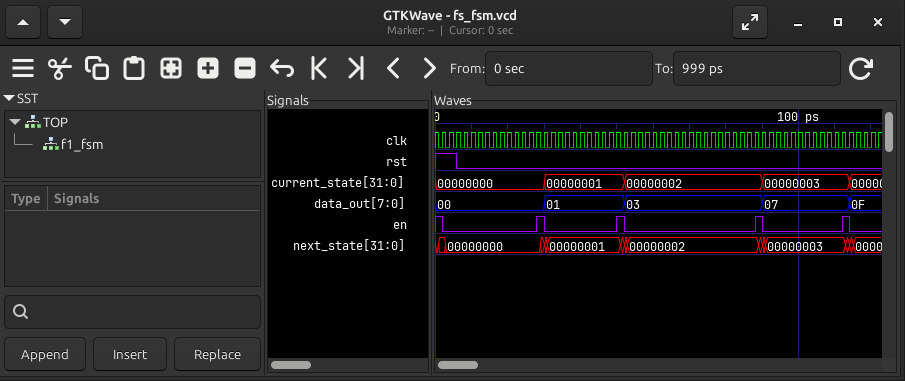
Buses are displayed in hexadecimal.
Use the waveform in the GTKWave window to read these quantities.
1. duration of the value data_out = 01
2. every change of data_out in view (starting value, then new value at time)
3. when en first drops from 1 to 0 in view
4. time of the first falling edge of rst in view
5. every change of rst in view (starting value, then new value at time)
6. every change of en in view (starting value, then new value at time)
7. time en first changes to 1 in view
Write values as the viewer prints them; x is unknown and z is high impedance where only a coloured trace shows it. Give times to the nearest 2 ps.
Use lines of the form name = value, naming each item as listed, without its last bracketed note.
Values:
duration of the value data_out = 01 = 22 ps
every change of data_out in view = 00, 01 at 30 ps, 03 at 52 ps, 07 at 90 ps, 0F at 114 ps
when en first drops from 1 to 0 in view = 2 ps
time of the first falling edge of rst in view = 6 ps
every change of rst in view = 1, 0 at 6 ps
every change of en in view = 1, 0 at 2 ps, 1 at 28 ps, 0 at 30 ps, 1 at 50 ps, 0 at 52 ps, 1 at 88 ps, 0 at 90 ps, 1 at 112 ps, 0 at 114 ps
time en first changes to 1 in view = 28 ps
